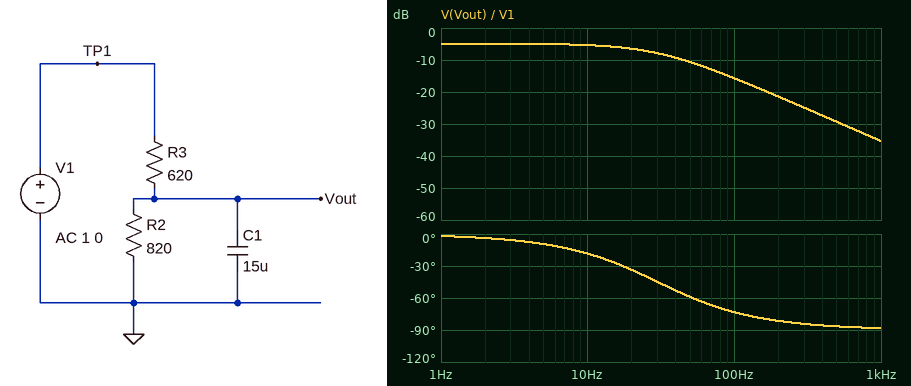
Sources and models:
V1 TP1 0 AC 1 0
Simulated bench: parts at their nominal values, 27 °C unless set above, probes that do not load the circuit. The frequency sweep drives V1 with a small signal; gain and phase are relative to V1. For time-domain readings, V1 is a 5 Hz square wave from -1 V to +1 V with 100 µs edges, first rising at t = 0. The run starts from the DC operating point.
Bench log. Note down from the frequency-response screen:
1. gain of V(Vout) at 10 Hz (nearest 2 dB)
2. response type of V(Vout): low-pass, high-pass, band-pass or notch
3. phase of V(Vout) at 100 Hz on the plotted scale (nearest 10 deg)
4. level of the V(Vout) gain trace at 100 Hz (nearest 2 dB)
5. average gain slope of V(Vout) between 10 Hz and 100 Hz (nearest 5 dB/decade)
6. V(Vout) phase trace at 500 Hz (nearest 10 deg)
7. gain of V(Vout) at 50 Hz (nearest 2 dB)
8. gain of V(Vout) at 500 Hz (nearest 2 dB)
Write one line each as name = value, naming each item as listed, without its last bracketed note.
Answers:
gain of V(Vout) at 10 Hz = -6 dB
response type of V(Vout): low-pass, high-pass, band-pass or notch = low-pass
phase of V(Vout) at 100 Hz on the plotted scale = -70 deg
level of the V(Vout) gain trace at 100 Hz = -16 dB
average gain slope of V(Vout) between 10 Hz and 100 Hz = -10 dB/decade
V(Vout) phase trace at 500 Hz = -90 deg
gain of V(Vout) at 50 Hz = -10 dB
gain of V(Vout) at 500 Hz = -30 dB
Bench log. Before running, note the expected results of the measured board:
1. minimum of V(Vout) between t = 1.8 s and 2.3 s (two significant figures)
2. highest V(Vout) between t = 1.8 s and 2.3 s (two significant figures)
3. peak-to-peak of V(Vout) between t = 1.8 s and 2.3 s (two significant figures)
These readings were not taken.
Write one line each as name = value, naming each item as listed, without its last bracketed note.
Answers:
minimum of V(Vout) between t = 1.8 s and 2.3 s = -570 mV
highest V(Vout) between t = 1.8 s and 2.3 s = 570 mV
peak-to-peak of V(Vout) between t = 1.8 s and 2.3 s = 1.1 V
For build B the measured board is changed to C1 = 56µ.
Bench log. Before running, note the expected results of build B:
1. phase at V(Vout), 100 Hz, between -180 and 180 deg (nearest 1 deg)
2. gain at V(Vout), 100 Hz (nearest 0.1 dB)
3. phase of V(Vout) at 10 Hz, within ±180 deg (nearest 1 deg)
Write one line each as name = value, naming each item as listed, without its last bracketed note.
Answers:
phase at V(Vout), 100 Hz, between -180 and 180 deg = -85 deg
gain at V(Vout), 100 Hz = -26.8 dB
phase of V(Vout) at 10 Hz, within ±180 deg = -51 deg
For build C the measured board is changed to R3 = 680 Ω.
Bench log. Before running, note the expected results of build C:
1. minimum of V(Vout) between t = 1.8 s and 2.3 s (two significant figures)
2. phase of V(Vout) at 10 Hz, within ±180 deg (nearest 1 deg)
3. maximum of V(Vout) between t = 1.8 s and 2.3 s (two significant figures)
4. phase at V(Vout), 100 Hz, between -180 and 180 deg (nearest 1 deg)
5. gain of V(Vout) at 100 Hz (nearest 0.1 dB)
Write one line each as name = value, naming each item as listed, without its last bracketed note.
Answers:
minimum of V(Vout) between t = 1.8 s and 2.3 s = -550 mV
phase of V(Vout) at 10 Hz, within ±180 deg = -19 deg
maximum of V(Vout) between t = 1.8 s and 2.3 s = 550 mV
phase at V(Vout), 100 Hz, between -180 and 180 deg = -74 deg
gain of V(Vout) at 100 Hz = -16.5 dB
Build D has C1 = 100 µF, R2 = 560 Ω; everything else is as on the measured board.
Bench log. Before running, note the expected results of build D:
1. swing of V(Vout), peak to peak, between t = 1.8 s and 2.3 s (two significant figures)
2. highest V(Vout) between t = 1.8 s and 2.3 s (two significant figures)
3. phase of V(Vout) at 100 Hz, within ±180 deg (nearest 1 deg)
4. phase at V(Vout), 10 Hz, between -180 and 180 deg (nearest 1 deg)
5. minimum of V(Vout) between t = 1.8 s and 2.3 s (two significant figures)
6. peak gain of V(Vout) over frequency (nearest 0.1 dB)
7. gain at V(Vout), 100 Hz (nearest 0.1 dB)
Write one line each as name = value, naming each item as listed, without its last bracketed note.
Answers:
swing of V(Vout), peak to peak, between t = 1.8 s and 2.3 s = 890 mV
highest V(Vout) between t = 1.8 s and 2.3 s = 440 mV
phase of V(Vout) at 100 Hz, within ±180 deg = -87 deg
phase at V(Vout), 10 Hz, between -180 and 180 deg = -62 deg
minimum of V(Vout) between t = 1.8 s and 2.3 s = -440 mV
peak gain of V(Vout) over frequency = -6.5 dB
gain at V(Vout), 100 Hz = -31.8 dB
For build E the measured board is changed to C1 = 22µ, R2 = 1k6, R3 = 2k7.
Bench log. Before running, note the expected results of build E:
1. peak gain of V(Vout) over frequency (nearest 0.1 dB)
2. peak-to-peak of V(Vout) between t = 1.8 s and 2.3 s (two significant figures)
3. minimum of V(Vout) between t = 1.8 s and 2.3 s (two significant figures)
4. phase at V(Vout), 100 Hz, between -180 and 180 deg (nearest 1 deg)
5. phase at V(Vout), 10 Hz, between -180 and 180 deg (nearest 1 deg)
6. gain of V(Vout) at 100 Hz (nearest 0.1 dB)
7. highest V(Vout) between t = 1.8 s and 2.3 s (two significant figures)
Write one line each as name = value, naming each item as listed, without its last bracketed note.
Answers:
peak gain of V(Vout) over frequency = -8.6 dB
peak-to-peak of V(Vout) between t = 1.8 s and 2.3 s = 730 mV
minimum of V(Vout) between t = 1.8 s and 2.3 s = -360 mV
phase at V(Vout), 100 Hz, between -180 and 180 deg = -86 deg
phase at V(Vout), 10 Hz, between -180 and 180 deg = -54 deg
gain of V(Vout) at 100 Hz = -31.5 dB
highest V(Vout) between t = 1.8 s and 2.3 s = 360 mV
